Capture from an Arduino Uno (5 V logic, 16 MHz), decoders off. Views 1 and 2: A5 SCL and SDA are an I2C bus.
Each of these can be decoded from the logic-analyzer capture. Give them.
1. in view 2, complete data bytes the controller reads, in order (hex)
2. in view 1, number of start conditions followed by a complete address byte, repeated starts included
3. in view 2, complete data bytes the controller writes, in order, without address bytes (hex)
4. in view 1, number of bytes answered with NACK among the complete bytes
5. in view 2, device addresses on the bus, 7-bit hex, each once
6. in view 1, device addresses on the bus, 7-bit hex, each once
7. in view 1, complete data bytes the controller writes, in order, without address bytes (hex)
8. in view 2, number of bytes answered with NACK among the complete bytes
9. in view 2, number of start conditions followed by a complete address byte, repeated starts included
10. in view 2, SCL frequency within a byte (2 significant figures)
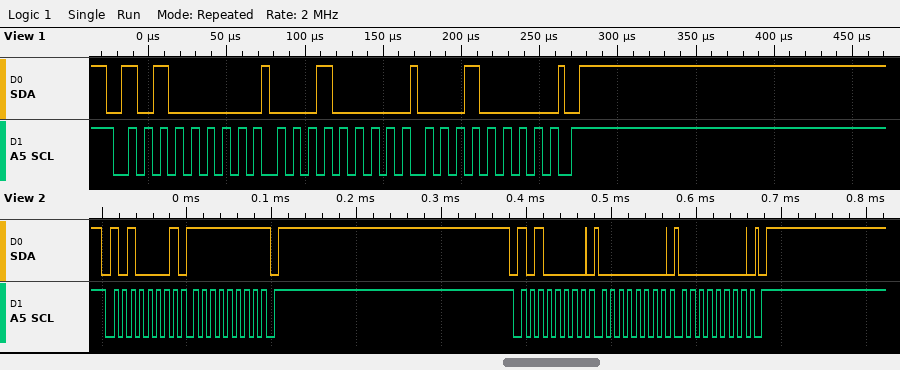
FF
1
00 00
0
0x50
0x50
10 10
1
2
100 kHz
